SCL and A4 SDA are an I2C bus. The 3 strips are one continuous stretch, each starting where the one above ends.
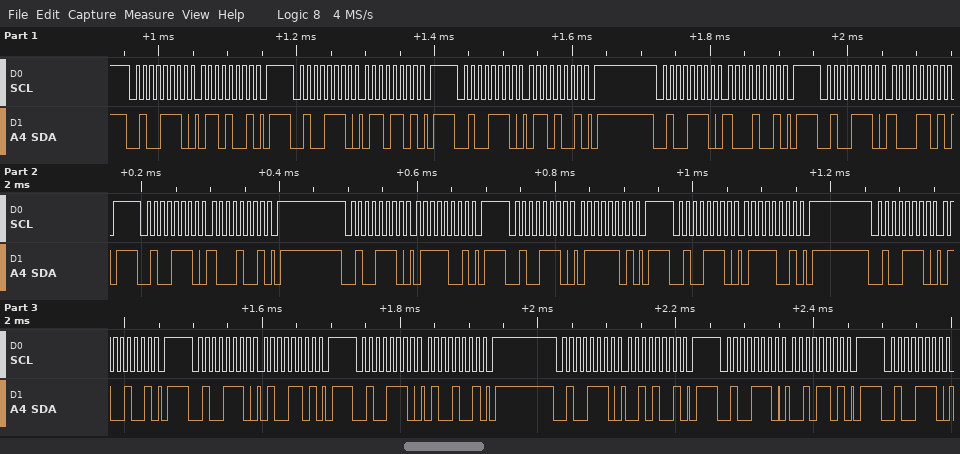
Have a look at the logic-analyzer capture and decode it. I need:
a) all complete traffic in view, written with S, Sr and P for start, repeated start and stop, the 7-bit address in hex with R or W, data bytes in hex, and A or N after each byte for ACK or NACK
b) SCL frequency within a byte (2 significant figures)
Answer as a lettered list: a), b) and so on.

a) S 27W A 69 A P S 27W A 6D A P S 27W A 69 A P S 27W A 89 A P S 27W A 8D A P S 27W A 89 A P S 27W A 79 A P S 27W A 7D A P S 27W A 79 A P S 27W A 49 A P S 27W A 4D A P S 27W A 49 A P S 27W A 29 A P S 27W A 2D A P S 27W A
b) 100 kHz
